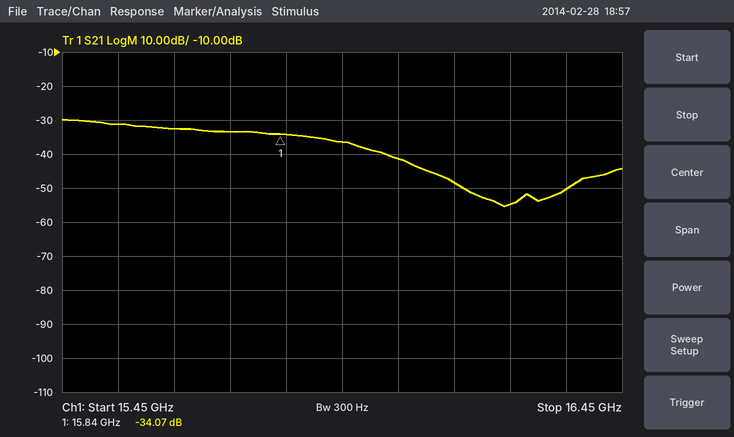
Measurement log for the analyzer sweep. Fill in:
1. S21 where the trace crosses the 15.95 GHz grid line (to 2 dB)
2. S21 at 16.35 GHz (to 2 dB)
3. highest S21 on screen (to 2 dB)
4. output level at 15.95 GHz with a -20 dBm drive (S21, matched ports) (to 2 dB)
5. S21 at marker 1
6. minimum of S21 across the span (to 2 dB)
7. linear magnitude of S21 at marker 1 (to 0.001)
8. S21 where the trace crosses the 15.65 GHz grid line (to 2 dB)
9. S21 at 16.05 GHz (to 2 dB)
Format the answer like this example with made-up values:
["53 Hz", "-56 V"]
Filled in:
["-36 dB", "-50 dB", "-30 dB", "-56 dBm", "-34.07 dB", "-56 dB", "0.020", "-32 dB", "-42 dB"]
